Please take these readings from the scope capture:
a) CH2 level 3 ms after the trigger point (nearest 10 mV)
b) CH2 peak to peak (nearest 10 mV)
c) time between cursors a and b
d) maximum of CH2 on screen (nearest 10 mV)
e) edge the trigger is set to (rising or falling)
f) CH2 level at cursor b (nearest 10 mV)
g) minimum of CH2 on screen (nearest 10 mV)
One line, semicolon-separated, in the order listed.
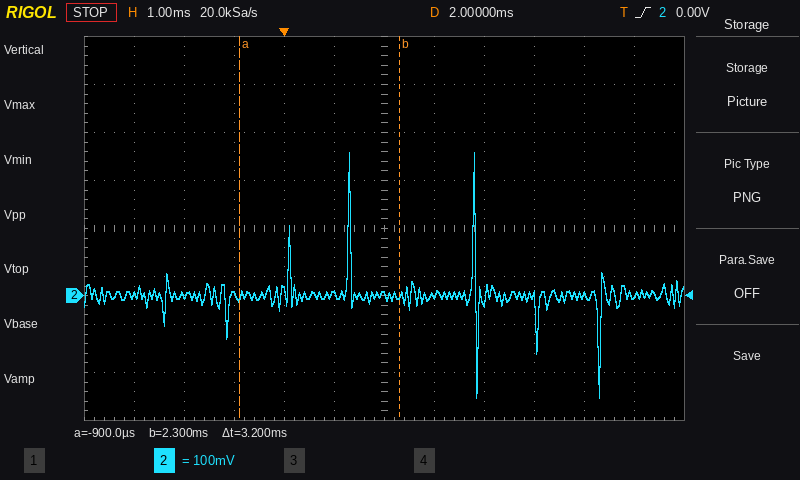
0 mV; 510 mV; 3.2 ms; 300 mV; rising; 0 mV; -210 mV
